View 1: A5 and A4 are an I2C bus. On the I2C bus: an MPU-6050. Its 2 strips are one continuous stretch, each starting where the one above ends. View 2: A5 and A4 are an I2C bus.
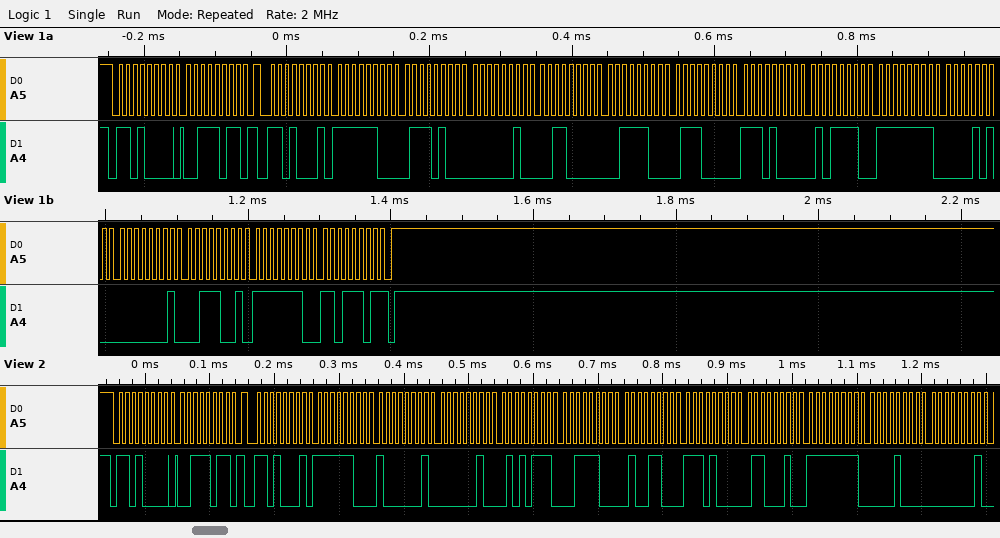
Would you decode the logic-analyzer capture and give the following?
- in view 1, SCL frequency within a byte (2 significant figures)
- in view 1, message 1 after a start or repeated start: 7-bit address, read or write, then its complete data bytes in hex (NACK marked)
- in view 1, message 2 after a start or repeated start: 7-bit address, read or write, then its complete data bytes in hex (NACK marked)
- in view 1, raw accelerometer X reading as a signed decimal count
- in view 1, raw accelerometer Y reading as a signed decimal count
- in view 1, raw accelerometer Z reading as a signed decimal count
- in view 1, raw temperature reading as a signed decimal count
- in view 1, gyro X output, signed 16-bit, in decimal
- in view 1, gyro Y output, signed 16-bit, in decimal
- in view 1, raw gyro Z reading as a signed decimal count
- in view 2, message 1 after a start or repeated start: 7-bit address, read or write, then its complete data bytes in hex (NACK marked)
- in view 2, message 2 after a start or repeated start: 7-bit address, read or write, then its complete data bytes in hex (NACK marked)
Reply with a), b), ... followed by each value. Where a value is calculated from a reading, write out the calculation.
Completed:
a) 100 kHz
b) 0x68 write: 3B
c) 0x68 read: FC 74 02 30 3C 70 E8 5E FF 0A 01 39 FE DD NACK
d) 0xFC74 = -908
e) 0x0230 = 560
f) 0x3C70 = 15472
g) 0xE85E = -6050
h) 0xFF0A = -246
i) 0x0139 = 313
j) 0xFEDD = -291
k) 0x68 write: 3B
l) 0x68 read: FC 81 02 57 3C 4C E8 62 FF 08 01
